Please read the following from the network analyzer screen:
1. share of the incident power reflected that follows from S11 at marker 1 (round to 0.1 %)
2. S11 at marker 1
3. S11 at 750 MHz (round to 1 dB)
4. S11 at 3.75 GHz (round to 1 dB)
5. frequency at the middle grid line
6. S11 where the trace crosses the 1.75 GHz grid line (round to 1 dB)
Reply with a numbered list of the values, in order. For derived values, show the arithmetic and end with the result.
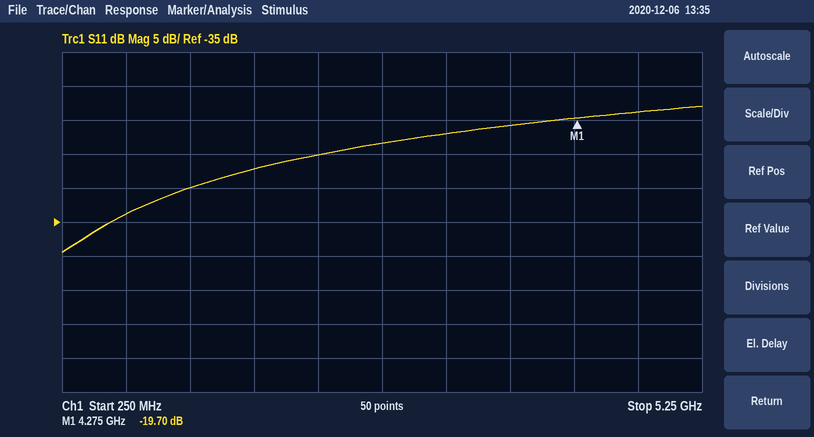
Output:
1. 10^(-19.7/10) ≈ 1.1 %
2. -19.70 dB
3. -34 dB
4. -21 dB
5. 2.75 GHz
6. -27 dB
